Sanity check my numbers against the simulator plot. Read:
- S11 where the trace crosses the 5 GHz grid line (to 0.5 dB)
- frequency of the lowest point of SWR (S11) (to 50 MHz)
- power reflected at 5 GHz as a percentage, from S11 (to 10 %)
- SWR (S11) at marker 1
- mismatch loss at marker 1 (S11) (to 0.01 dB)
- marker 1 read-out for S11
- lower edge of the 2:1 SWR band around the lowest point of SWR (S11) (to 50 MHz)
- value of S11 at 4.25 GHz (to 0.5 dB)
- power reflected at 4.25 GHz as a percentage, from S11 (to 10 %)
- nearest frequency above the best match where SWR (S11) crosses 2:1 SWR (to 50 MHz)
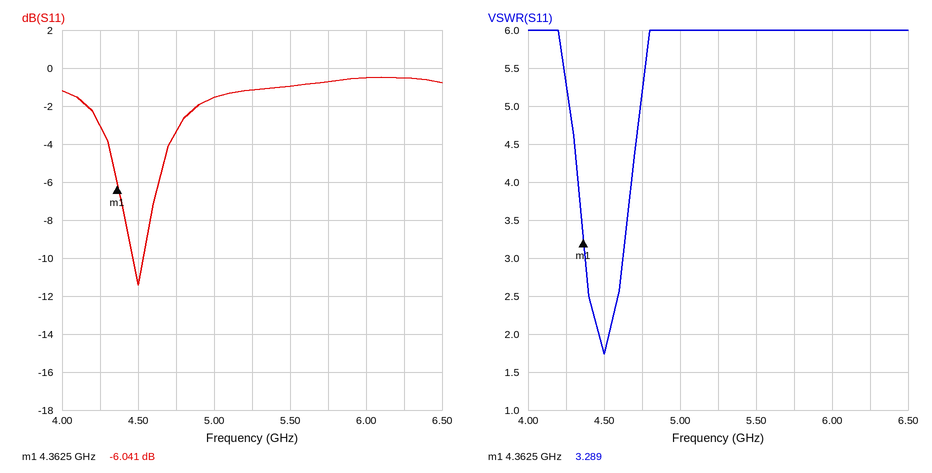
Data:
-1.5 dB
4.50 GHz
70 %
3.289
1.24 dB
-6.041 dB
4.45 GHz
-3.0 dB
50 %
4.55 GHz
